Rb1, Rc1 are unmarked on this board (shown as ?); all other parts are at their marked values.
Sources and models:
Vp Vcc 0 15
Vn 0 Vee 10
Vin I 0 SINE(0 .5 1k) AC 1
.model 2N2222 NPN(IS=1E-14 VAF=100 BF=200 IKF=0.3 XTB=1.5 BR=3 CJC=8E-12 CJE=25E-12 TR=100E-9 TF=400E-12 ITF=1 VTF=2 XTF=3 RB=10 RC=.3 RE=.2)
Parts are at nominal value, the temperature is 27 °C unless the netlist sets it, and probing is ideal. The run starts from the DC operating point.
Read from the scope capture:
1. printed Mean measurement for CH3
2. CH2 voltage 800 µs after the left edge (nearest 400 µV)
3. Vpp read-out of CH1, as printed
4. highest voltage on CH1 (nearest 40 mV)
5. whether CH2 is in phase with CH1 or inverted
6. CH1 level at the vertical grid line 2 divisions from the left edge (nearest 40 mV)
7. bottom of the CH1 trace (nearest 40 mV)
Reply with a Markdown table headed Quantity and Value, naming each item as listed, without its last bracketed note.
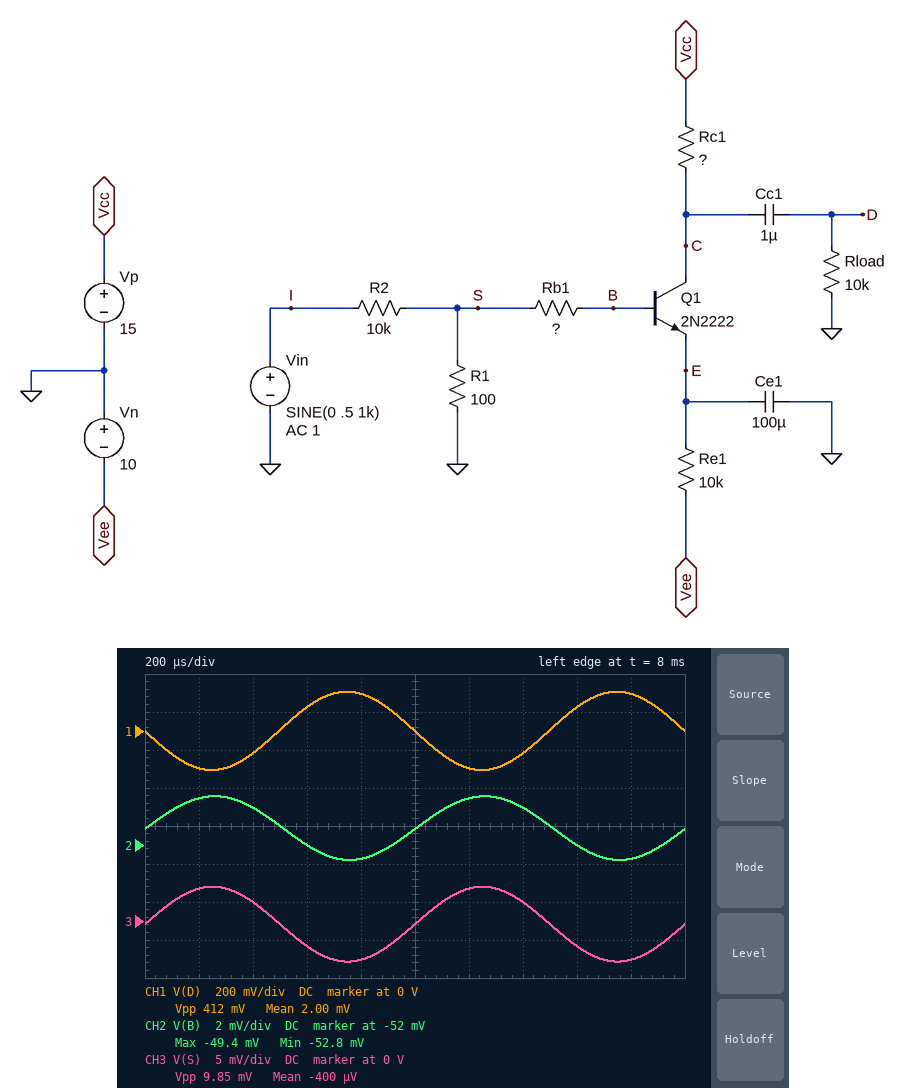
| Quantity | Value |
|---|---|
| printed Mean measurement for CH3 | -400 µV |
| CH2 voltage 800 µs after the left edge | -52.8 mV |
| Vpp read-out of CH1, as printed | 412 mV |
| highest voltage on CH1 | 200 mV |
| whether CH2 is in phase with CH1 or inverted | inverted |
| CH1 level at the vertical grid line 2 divisions from the left edge | -120 mV |
| bottom of the CH1 trace | -200 mV |
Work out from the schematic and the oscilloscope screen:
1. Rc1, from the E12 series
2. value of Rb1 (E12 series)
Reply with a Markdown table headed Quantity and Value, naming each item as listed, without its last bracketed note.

| Quantity | Value |
|---|---|
| Rc1, from the E12 series | 5.6 kΩ |
| value of Rb1 | 12 kΩ |
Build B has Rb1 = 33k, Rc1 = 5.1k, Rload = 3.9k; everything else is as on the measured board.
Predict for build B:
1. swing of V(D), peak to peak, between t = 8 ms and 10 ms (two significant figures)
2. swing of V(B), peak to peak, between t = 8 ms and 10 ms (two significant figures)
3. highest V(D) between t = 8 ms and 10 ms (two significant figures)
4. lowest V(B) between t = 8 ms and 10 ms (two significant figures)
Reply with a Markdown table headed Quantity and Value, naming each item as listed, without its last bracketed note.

| Quantity | Value |
|---|---|
| swing of V(D), peak to peak, between t = 8 ms and 10 ms | 120 mV |
| swing of V(B), peak to peak, between t = 8 ms and 10 ms | 1.6 mV |
| highest V(D) between t = 8 ms and 10 ms | 60 mV |
| lowest V(B) between t = 8 ms and 10 ms | -140 mV |
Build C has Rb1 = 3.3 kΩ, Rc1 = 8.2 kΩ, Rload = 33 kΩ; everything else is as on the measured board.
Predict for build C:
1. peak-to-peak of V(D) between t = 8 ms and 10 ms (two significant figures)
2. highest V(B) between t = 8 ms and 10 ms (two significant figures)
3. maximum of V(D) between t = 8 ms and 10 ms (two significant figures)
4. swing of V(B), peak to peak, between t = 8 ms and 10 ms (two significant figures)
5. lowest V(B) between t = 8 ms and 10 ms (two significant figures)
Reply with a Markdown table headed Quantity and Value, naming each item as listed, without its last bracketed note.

| Quantity | Value |
|---|---|
| peak-to-peak of V(D) between t = 8 ms and 10 ms | 1.4 V |
| highest V(B) between t = 8 ms and 10 ms | -12 mV |
| maximum of V(D) between t = 8 ms and 10 ms | 690 mV |
| swing of V(B), peak to peak, between t = 8 ms and 10 ms | 6.3 mV |
| lowest V(B) between t = 8 ms and 10 ms | -18 mV |
